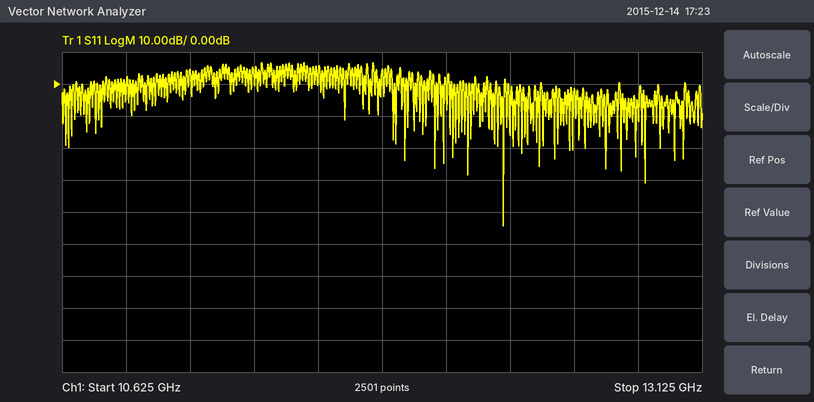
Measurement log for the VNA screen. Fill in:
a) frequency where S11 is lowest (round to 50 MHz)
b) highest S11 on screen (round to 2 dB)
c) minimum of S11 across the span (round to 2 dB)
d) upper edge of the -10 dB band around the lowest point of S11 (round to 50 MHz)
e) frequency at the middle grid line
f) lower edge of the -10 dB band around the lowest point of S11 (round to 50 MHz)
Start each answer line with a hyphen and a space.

- 12.35 GHz
- 6 dB
- -44 dB
- 12.35 GHz
- 11.875 GHz
- 12.35 GHz
